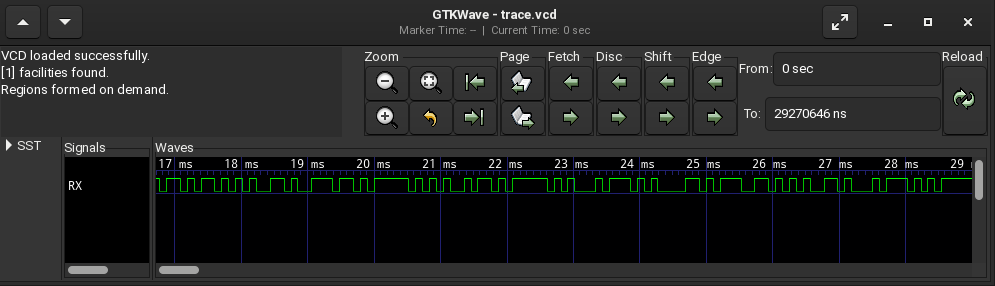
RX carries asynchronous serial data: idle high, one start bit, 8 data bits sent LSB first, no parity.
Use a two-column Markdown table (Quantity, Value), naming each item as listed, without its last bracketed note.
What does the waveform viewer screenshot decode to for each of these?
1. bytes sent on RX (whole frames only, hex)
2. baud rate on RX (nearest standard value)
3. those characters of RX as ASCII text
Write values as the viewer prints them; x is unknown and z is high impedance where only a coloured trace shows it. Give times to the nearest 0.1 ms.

| Quantity | Value |
|---|---|
| bytes sent on RX | 6B, 65, 6E, 5F, 69, 5F, 74, 61, 67, 65, 74 |
| baud rate on RX | 9600 baud |
| those characters of RX as ASCII text | "ken_i_taget" |
